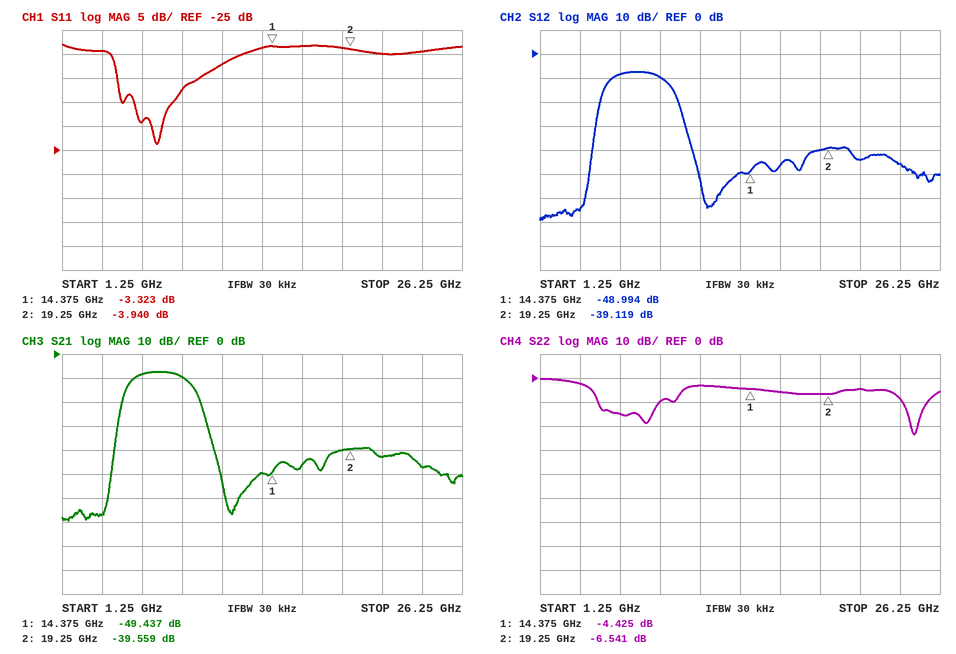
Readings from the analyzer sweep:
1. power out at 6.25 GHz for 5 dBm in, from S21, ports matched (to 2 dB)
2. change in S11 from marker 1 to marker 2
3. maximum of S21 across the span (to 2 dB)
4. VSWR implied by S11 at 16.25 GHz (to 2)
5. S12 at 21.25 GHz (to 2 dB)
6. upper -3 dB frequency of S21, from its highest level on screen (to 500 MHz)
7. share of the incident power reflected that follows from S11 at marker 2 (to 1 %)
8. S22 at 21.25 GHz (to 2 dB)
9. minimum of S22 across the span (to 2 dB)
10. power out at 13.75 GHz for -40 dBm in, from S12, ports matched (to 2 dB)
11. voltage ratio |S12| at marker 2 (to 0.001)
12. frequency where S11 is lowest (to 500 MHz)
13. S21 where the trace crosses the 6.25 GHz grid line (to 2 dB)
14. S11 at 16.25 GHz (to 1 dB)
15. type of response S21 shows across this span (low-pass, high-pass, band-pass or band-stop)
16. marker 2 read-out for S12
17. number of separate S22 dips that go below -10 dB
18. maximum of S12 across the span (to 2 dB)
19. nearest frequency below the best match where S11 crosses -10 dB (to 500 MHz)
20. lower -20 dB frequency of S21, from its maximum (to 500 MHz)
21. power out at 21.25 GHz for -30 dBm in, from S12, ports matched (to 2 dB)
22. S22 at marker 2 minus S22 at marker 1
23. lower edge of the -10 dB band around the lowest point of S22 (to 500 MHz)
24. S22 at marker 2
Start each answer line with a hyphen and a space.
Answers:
- -4 dBm
- -0.617 dB
- -8 dB
- 6
- -44 dB
- 9.0 GHz
- 40 %
- -4 dB
- -24 dB
- -90 dBm
- 0.011
- 7.0 GHz
- -8 dB
- -3 dB
- band-pass
- -39.119 dB
- 2
- -8 dB
- 4.5 GHz
- 5.0 GHz
- -74 dBm
- -2.116 dB
- 24.0 GHz
- -6.541 dB
